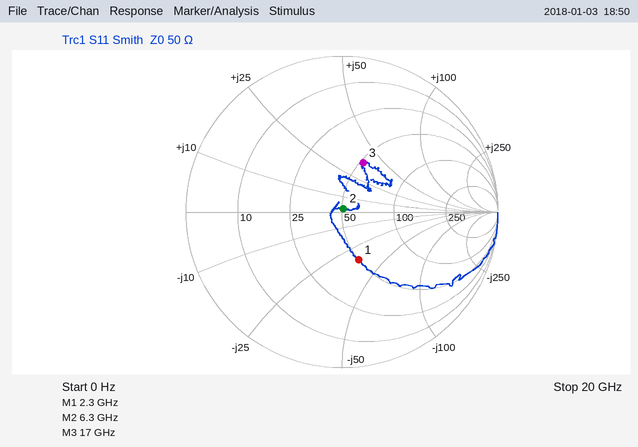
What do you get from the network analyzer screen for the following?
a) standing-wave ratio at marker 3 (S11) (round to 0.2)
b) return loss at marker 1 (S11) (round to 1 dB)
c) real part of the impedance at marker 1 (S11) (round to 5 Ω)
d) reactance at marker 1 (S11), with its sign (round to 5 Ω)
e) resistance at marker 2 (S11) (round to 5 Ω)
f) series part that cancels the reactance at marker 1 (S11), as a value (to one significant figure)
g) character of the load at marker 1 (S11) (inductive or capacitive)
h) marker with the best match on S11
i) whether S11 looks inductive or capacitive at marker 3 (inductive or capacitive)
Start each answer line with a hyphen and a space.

- 2.0
- 10 dB
- 50 Ω
- -35 Ω
- 50 Ω
- 2 nH
- capacitive
- marker 2
- inductive
